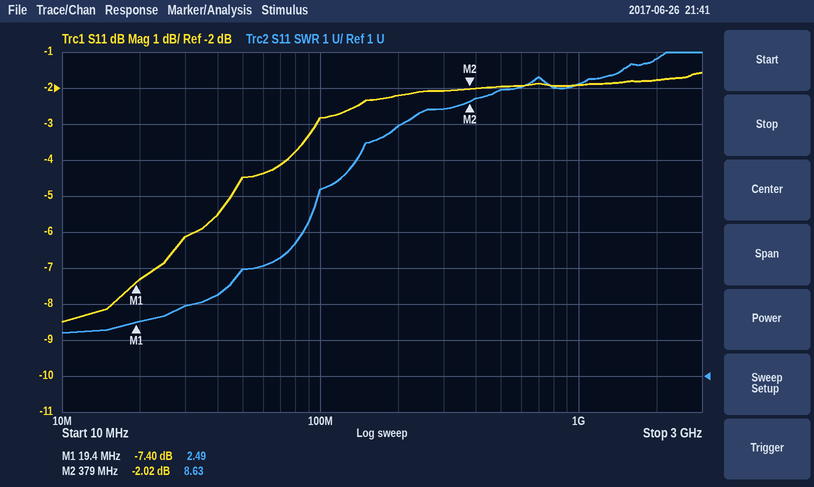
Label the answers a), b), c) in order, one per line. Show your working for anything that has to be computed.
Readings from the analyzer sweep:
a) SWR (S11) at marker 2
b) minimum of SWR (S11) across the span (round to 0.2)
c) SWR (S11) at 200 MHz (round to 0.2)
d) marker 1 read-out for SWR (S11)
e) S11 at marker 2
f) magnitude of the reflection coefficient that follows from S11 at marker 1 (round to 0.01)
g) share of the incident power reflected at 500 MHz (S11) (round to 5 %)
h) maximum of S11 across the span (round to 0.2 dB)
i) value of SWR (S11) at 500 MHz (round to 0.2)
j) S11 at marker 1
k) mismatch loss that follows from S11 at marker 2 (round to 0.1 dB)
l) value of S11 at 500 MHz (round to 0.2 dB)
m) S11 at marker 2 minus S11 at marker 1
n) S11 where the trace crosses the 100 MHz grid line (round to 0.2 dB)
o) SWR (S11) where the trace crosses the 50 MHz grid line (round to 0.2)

a) 8.63
b) 2.2
c) 8.0
d) 2.49
e) -2.02 dB
f) 10^(-7.4/20) ≈ 0.43
g) 10^(-2/10) ≈ 63.1 %, so 65 % to the nearest 5 %
h) -1.6 dB
i) 9.0
j) -7.40 dB
k) −10 log10(1 − 10^(-2.02/10)) ≈ 4.3 dB
l) -2.0 dB
m) -2.02 − (-7.4) = 5.38 dB
n) -2.8 dB
o) 4.0
